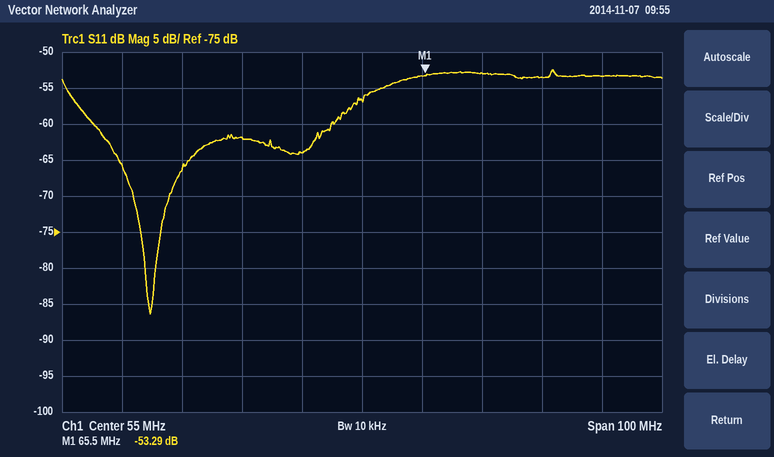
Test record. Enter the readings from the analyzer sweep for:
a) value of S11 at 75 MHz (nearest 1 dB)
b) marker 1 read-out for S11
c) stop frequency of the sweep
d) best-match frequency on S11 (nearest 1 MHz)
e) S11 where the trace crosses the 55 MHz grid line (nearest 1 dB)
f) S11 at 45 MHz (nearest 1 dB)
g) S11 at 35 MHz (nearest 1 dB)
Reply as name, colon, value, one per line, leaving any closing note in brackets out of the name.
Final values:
value of S11 at 75 MHz: -53 dB
marker 1 read-out for S11: -53.29 dB
stop frequency of the sweep: 105 MHz
best-match frequency on S11: 20 MHz
S11 where the trace crosses the 55 MHz grid line: -57 dB
S11 at 45 MHz: -64 dB
S11 at 35 MHz: -62 dB
